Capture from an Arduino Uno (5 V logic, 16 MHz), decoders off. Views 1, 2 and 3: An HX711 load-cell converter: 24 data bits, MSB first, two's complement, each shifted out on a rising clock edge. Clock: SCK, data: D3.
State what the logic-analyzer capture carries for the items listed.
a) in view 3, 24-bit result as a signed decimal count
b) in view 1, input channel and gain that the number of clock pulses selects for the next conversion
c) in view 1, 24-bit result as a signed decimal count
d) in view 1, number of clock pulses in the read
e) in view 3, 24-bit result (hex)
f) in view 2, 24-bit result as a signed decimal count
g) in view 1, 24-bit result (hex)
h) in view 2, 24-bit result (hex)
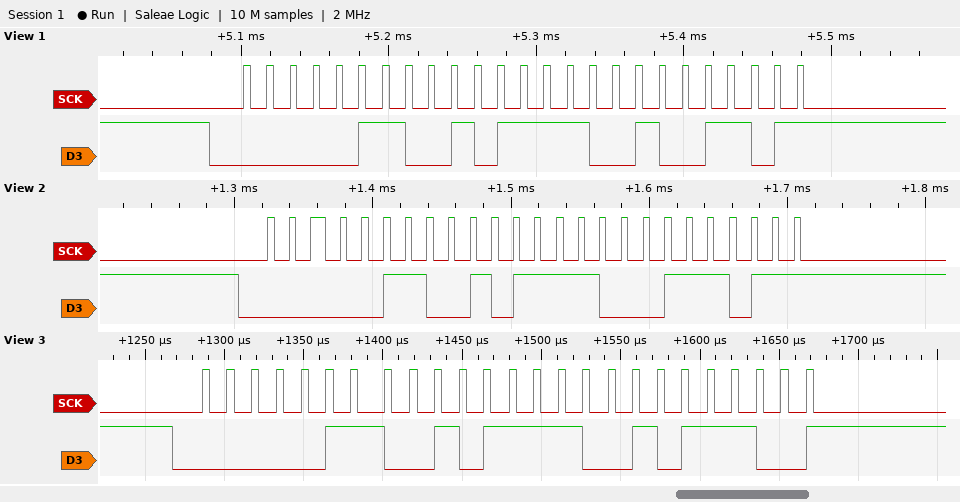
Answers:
417372
channel A, gain 128
417357
25
0x065E5C
417339
0x065E4D
0x065E3B
